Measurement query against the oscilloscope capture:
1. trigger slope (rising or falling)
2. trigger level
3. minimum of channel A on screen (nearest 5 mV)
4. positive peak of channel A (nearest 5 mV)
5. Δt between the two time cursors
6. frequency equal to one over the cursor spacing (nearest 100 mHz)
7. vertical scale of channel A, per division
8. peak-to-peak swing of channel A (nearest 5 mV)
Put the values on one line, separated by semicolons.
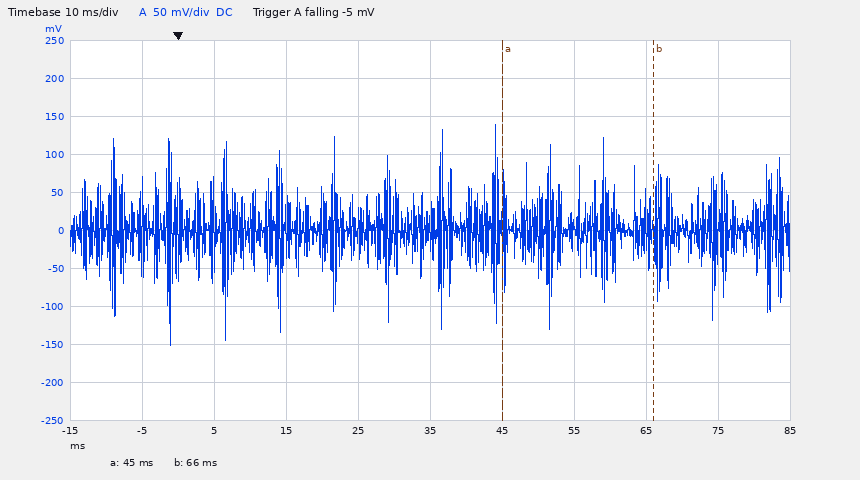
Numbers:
falling; -5 mV; -150 mV; 140 mV; 21 ms; 47.6 Hz; 50 mV; 290 mV
